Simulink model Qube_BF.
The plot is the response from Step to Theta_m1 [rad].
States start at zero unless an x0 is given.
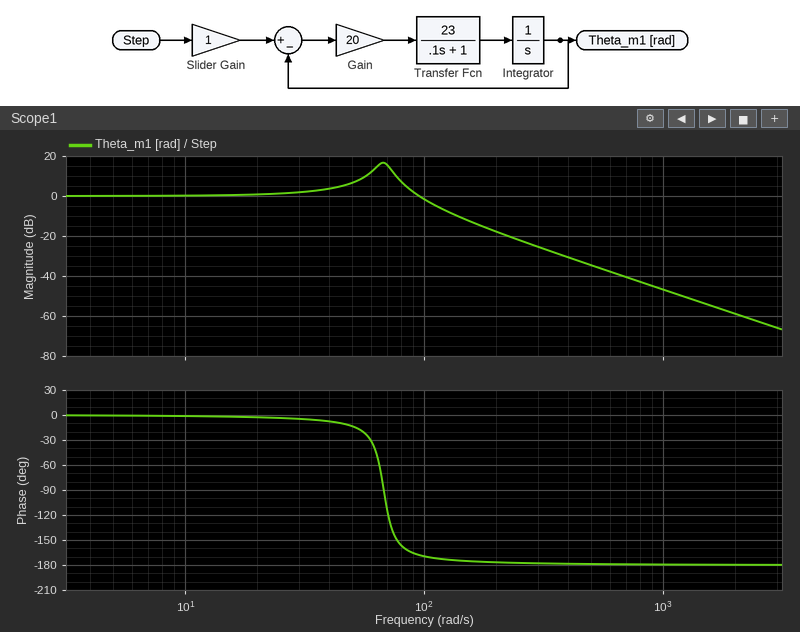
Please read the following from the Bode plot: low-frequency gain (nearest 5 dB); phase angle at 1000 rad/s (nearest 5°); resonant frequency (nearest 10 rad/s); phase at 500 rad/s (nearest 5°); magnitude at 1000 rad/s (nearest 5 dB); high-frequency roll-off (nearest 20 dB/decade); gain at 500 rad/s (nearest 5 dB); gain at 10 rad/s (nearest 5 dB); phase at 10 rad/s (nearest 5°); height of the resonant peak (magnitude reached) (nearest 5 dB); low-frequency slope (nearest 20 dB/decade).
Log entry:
0 dB
-180°
70 rad/s
-180°
-45 dB
-40 dB/decade
-35 dB
0 dB
0°
15 dB
0 dB/decade
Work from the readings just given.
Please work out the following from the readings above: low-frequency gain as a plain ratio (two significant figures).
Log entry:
1.0
